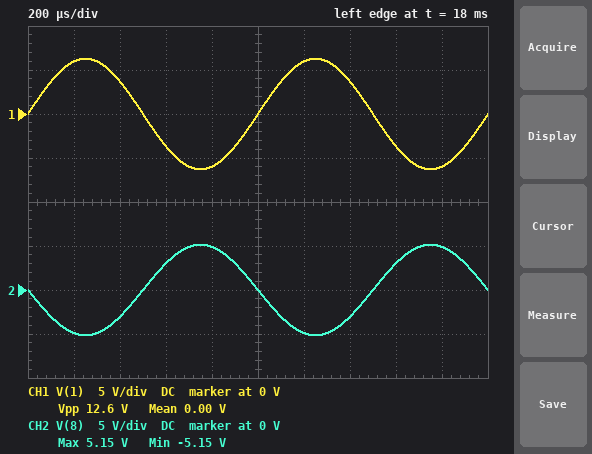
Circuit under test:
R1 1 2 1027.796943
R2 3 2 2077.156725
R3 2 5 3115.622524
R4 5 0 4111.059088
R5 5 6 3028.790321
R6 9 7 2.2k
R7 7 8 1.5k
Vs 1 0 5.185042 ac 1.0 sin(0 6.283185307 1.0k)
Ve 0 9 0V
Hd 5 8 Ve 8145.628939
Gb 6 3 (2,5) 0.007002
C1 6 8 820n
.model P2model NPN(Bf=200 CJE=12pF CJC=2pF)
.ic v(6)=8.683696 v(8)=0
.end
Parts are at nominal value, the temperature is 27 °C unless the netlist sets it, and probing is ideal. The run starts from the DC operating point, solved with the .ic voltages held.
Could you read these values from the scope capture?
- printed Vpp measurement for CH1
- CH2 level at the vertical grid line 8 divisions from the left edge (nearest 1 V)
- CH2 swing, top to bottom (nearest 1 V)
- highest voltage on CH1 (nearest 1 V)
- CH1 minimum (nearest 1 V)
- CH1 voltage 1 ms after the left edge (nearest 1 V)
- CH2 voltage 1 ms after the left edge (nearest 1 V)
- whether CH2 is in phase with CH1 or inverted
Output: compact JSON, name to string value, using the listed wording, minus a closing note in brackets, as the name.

{"printed Vpp measurement for CH1": "12.6 V", "CH2 level at the vertical grid line 8 divisions from the left edge": "3 V", "CH2 swing, top to bottom": "10 V", "highest voltage on CH1": "6 V", "CH1 minimum": "-6 V", "CH1 voltage 1 ms after the left edge": "0 V", "CH2 voltage 1 ms after the left edge": "0 V", "whether CH2 is in phase with CH1 or inverted": "inverted"}
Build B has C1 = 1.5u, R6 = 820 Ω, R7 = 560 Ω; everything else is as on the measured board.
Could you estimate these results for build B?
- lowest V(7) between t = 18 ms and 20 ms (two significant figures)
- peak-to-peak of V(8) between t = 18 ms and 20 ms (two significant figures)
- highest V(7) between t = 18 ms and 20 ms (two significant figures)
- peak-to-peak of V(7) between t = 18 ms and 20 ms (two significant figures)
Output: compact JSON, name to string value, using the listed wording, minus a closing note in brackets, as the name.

{"lowest V(7) between t = 18 ms and 20 ms": "-700 mV", "peak-to-peak of V(8) between t = 18 ms and 20 ms": "2.4 V", "highest V(7) between t = 18 ms and 20 ms": "700 mV", "peak-to-peak of V(7) between t = 18 ms and 20 ms": "1.4 V"}
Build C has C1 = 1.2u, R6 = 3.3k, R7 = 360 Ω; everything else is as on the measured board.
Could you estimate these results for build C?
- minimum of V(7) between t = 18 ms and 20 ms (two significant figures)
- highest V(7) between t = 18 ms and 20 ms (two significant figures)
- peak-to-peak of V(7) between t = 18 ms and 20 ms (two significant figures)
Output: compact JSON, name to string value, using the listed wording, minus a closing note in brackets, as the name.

{"minimum of V(7) between t = 18 ms and 20 ms": "-4.5 V", "highest V(7) between t = 18 ms and 20 ms": "4.5 V", "peak-to-peak of V(7) between t = 18 ms and 20 ms": "9.1 V"}
